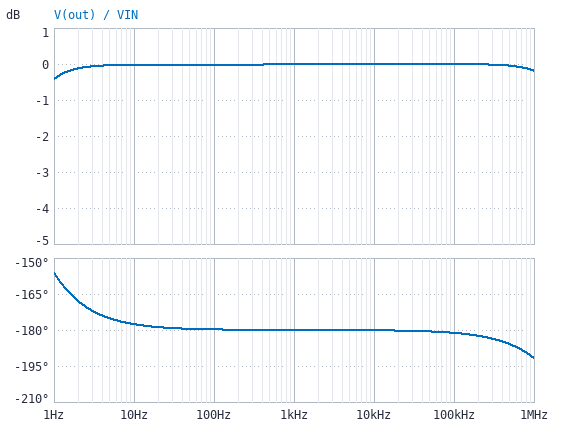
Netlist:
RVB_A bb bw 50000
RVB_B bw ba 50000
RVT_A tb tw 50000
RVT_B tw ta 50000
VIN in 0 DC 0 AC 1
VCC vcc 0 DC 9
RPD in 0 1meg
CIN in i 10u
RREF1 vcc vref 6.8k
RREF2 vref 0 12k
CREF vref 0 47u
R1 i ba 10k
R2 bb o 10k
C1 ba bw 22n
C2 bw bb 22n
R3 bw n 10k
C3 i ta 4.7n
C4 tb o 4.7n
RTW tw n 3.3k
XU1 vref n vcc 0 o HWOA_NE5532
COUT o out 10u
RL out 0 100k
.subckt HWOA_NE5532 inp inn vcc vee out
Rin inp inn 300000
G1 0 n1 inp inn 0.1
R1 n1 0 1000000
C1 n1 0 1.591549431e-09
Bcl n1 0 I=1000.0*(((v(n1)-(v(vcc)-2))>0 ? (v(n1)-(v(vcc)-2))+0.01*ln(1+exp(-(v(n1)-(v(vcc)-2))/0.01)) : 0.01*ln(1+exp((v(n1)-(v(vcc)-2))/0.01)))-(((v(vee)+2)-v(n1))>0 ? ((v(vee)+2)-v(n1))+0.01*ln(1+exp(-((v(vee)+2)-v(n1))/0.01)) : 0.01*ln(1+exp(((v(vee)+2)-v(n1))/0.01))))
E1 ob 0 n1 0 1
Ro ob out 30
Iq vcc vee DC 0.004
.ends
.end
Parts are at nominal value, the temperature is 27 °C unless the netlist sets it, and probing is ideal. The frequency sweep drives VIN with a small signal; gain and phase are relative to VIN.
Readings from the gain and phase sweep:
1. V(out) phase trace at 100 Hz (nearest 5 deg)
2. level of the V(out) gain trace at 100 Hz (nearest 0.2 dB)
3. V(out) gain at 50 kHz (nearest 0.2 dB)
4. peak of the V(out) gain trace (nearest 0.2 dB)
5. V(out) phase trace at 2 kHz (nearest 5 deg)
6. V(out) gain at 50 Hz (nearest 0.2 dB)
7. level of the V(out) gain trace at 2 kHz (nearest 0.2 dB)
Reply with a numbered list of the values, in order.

1. -180 deg
2. 0 dB
3. 0 dB
4. 0 dB
5. -180 deg
6. 0 dB
7. 0 dB
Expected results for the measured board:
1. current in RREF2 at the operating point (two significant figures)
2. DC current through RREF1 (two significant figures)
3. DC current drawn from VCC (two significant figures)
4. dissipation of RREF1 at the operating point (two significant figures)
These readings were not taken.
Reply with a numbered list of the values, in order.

1. 480 µA
2. 480 µA
3. 4.5 mA
4. 1.6 mW
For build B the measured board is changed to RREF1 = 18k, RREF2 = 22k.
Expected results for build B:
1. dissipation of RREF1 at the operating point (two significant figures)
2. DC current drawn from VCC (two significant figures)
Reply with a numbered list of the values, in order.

1. 910 µW
2. 4.2 mA
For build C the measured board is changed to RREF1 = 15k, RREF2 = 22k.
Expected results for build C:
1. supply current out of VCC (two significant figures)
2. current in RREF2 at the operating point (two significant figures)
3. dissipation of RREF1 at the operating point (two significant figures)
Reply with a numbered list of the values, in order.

1. 4.2 mA
2. 240 µA
3. 890 µW
